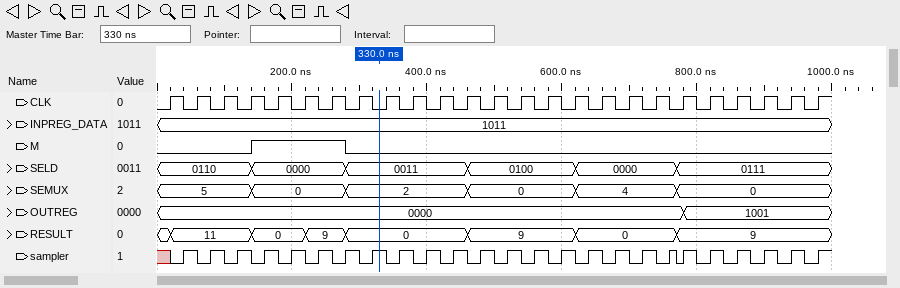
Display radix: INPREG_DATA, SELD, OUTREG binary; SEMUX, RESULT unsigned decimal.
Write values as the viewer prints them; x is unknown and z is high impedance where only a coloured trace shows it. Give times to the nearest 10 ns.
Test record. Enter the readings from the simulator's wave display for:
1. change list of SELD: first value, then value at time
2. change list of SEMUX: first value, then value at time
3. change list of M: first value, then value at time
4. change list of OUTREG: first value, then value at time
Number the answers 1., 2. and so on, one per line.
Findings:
1. 0110, 0000 at 140 ns, 0011 at 280 ns, 0100 at 460 ns, 0000 at 620 ns, 0111 at 770 ns
2. 5, 0 at 140 ns, 2 at 280 ns, 0 at 460 ns, 4 at 620 ns, 0 at 770 ns
3. 0, 1 at 140 ns, 0 at 280 ns
4. 0000, 1001 at 780 ns
